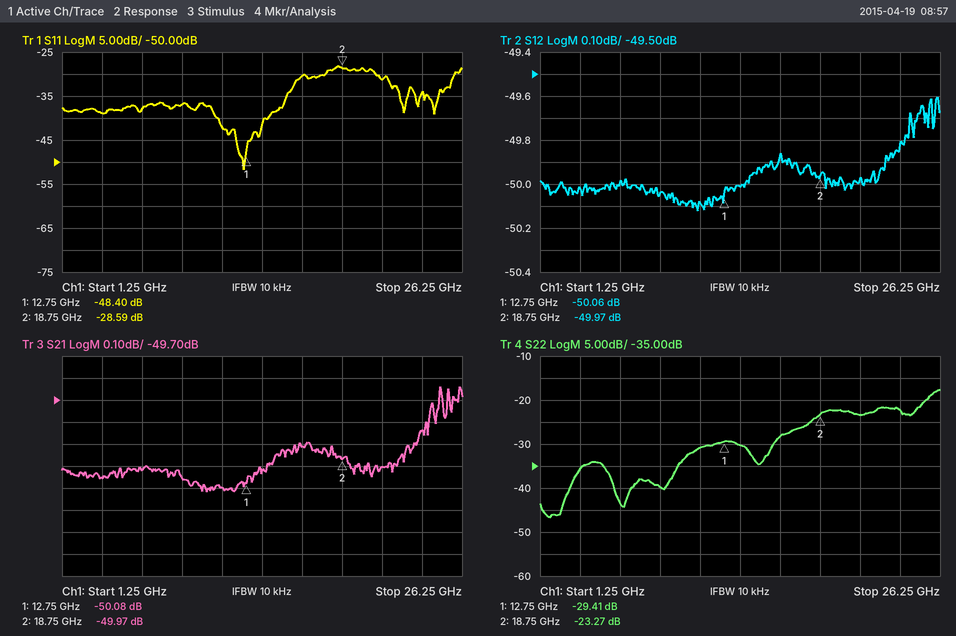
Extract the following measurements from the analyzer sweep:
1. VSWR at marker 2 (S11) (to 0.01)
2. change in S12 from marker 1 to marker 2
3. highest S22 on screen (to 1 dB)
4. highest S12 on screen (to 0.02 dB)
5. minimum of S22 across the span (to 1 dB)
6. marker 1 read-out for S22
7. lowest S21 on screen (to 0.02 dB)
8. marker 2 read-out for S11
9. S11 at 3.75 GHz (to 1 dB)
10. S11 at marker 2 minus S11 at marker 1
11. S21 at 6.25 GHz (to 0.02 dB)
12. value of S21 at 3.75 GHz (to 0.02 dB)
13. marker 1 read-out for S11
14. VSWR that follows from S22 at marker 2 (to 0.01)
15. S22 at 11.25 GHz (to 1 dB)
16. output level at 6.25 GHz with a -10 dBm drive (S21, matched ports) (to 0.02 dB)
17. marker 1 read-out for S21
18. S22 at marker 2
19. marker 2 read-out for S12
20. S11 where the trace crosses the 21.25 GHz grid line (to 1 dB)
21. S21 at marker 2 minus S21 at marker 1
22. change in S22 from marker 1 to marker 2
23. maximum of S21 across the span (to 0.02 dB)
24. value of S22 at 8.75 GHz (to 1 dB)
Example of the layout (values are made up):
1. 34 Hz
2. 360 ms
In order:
1. 1.08
2. 0.09 dB
3. -18 dB
4. -49.60 dB
5. -47 dB
6. -29.41 dB
7. -50.12 dB
8. -28.59 dB
9. -39 dB
10. 19.81 dB
11. -50.02 dB
12. -50.06 dB
13. -48.40 dB
14. 1.15
15. -31 dB
16. -60.02 dBm
17. -50.08 dB
18. -23.27 dB
19. -49.97 dB
20. -31 dB
21. 0.11 dB
22. 6.14 dB
23. -49.64 dB
24. -40 dB
